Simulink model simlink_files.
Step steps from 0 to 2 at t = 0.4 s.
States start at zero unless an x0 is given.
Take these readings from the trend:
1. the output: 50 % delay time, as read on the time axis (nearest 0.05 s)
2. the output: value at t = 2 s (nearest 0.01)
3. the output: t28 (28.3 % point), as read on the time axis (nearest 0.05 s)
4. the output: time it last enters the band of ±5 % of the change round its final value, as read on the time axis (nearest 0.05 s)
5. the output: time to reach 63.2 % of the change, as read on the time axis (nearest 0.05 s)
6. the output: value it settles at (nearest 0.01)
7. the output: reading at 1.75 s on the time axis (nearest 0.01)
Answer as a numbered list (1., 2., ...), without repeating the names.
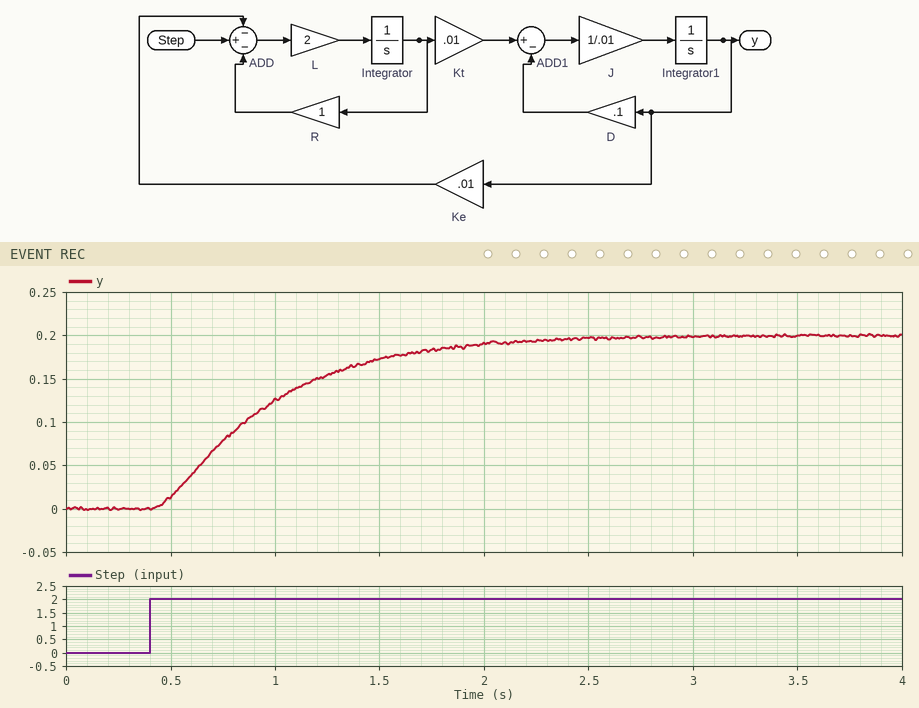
1. 0.85 s
2. 0.19
3. 0.65 s
4. 2.00 s
5. 1.00 s
6. 0.20
7. 0.18
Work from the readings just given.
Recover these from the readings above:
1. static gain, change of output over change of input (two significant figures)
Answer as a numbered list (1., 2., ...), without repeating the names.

1. 0.10
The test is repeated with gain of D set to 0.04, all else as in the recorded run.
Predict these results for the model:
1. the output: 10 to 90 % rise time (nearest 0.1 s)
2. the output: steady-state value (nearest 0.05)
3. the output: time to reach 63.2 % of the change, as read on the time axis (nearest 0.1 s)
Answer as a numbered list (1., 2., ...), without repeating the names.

1. 1.3 s
2. 0.50
3. 1.2 s
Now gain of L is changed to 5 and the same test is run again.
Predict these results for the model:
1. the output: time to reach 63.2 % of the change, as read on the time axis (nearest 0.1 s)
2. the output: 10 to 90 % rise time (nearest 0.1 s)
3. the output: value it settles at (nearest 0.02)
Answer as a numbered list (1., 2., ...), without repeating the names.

1. 0.7 s
2. 0.5 s
3. 0.20
